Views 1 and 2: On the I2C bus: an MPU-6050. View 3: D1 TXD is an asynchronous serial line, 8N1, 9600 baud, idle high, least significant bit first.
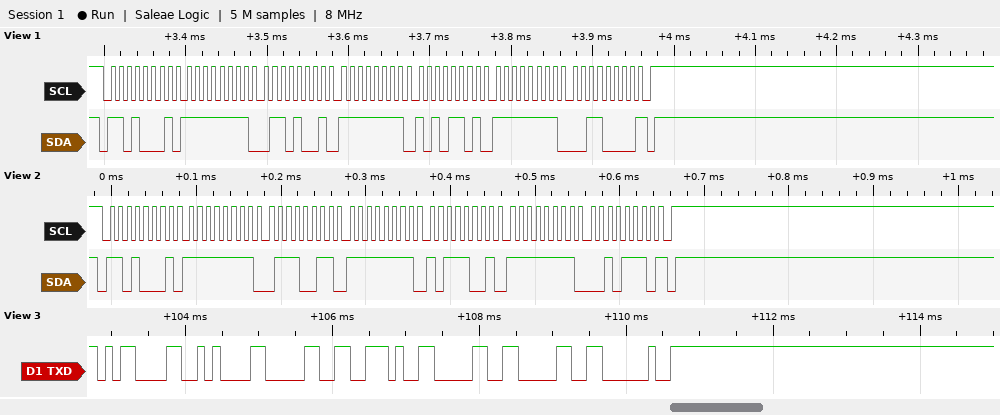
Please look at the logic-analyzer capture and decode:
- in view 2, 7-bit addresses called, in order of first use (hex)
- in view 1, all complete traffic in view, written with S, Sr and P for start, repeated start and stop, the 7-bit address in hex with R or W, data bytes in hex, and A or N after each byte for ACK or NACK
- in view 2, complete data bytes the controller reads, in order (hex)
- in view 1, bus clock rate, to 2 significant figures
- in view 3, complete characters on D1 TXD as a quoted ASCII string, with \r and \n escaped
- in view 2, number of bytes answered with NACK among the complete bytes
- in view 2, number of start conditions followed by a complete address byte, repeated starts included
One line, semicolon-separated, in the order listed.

0x68; S 68R A FF A 69 A FF A AD A FF A 30 N P; FF 73 FF B9 FF 2E; 100 kHz; "\r\n0.00 "; 1; 1
